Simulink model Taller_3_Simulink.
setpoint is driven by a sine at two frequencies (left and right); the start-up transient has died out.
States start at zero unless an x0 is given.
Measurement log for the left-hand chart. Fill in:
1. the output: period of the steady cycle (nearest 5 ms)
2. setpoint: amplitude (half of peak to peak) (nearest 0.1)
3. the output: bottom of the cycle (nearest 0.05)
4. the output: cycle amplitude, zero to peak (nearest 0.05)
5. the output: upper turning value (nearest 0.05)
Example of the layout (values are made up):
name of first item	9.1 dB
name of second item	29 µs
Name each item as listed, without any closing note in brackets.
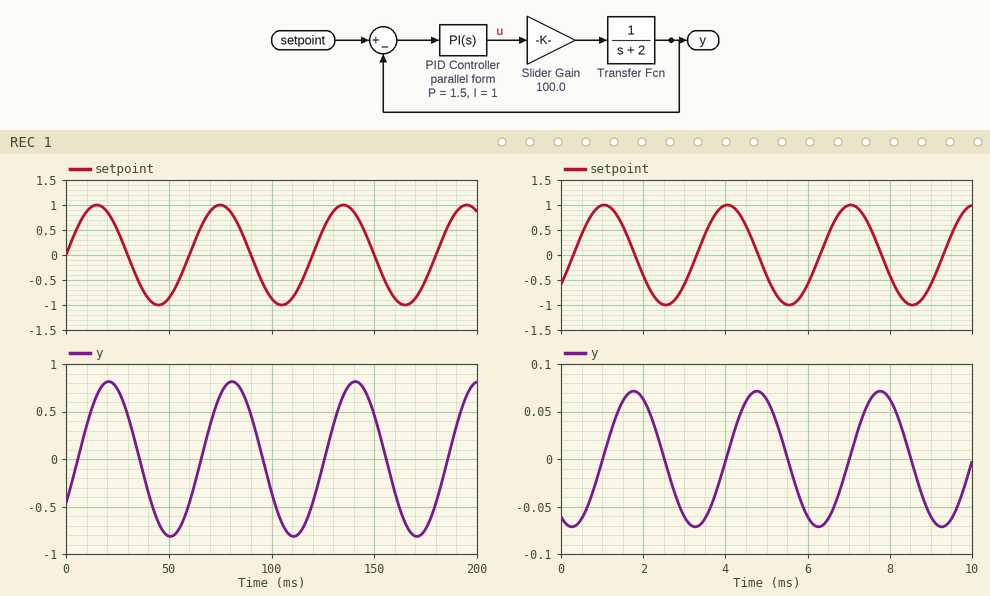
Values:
the output: period of the steady cycle	60 ms
setpoint: amplitude (half of peak to peak)	1.0
the output: bottom of the cycle	-0.80
the output: cycle amplitude, zero to peak	0.80
the output: upper turning value	0.80
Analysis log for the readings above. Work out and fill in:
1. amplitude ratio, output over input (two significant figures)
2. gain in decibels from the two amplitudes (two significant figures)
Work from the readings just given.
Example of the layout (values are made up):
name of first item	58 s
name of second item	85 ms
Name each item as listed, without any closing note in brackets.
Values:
amplitude ratio, output over input	0.80
gain in decibels from the two amplitudes	-1.9 dB
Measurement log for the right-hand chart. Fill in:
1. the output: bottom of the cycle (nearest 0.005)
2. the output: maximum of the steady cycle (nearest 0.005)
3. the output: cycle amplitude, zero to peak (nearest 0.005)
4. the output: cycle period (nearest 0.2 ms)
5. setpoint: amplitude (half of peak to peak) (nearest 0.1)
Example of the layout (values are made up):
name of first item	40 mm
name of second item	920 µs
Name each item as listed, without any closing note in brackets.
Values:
the output: bottom of the cycle	-0.070
the output: maximum of the steady cycle	0.070
the output: cycle amplitude, zero to peak	0.070
the output: cycle period	3.0 ms
setpoint: amplitude (half of peak to peak)	1.0
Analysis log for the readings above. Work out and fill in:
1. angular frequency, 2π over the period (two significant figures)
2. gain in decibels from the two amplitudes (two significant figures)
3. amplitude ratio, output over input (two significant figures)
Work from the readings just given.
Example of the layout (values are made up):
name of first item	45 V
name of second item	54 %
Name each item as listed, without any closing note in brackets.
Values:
angular frequency, 2π over the period	2.1 rad/ms
gain in decibels from the two amplitudes	-23 dB
amplitude ratio, output over input	0.070
